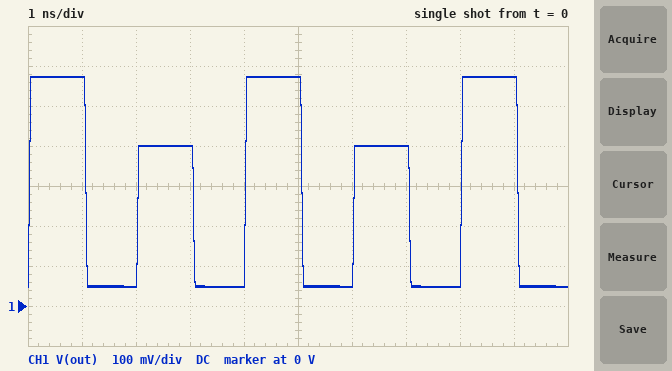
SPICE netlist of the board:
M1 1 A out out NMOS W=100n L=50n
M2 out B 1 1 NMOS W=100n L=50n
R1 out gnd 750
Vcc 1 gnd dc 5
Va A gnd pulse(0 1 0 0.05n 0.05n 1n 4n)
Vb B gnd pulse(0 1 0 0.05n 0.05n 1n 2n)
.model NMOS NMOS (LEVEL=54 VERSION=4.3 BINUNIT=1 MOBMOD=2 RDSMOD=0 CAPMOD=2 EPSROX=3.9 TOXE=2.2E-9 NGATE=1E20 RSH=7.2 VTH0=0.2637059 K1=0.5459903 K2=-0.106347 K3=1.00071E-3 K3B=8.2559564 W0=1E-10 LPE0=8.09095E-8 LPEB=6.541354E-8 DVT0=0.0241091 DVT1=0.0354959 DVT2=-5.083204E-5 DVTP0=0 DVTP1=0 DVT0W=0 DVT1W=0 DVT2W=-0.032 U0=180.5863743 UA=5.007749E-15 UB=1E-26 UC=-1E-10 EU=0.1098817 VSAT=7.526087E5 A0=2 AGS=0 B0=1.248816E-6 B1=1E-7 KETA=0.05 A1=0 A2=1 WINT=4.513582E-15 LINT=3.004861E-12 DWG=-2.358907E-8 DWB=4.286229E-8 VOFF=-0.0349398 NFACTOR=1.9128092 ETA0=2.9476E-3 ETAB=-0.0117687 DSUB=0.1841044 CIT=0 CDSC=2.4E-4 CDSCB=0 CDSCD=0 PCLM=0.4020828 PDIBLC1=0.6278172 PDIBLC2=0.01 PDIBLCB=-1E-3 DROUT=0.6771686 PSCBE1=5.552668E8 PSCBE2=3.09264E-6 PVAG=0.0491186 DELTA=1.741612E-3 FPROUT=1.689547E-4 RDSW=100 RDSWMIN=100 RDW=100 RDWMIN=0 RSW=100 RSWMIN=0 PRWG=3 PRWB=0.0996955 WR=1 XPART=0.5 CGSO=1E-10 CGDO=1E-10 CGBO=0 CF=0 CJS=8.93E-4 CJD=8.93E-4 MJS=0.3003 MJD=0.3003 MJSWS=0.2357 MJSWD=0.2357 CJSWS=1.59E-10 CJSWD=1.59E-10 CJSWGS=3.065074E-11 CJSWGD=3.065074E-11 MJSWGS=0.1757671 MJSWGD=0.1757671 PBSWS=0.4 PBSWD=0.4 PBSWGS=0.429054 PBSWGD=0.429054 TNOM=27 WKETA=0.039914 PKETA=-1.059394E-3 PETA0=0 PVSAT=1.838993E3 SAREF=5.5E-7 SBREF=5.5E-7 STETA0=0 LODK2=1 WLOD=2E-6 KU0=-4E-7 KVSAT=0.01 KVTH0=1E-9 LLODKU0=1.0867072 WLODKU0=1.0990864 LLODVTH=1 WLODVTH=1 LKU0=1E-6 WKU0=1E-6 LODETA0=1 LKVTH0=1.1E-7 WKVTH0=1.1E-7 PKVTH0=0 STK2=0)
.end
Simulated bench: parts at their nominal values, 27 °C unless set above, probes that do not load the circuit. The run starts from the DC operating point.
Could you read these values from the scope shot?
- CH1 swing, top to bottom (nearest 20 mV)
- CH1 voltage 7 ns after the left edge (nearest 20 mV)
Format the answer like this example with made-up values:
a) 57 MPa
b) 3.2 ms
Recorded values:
a) 520 mV
b) 400 mV
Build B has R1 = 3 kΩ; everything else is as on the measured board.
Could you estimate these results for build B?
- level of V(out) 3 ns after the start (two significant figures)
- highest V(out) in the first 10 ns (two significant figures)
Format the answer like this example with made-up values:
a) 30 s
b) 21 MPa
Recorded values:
a) 580 mV
b) 740 mV
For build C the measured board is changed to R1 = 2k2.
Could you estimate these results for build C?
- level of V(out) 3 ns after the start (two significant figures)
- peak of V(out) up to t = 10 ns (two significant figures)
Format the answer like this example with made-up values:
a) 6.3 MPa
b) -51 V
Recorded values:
a) 540 mV
b) 700 mV
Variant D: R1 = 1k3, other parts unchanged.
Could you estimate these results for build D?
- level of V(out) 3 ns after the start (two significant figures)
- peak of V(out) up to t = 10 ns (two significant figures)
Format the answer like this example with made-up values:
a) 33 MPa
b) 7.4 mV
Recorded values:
a) 480 mV
b) 640 mV
